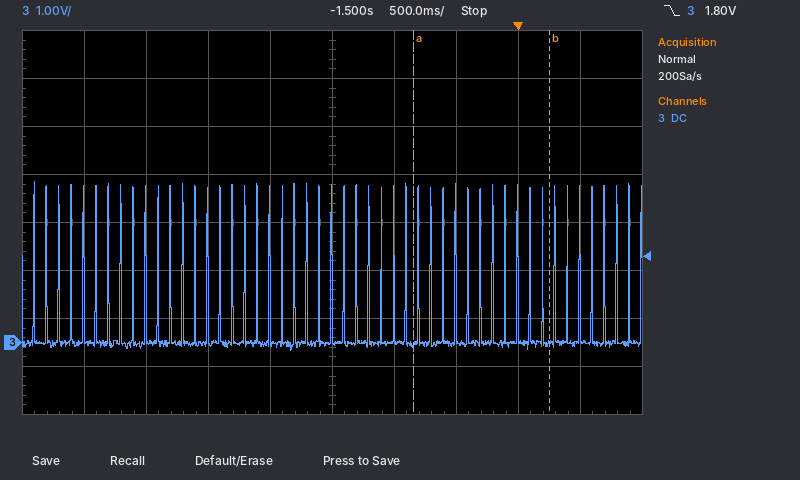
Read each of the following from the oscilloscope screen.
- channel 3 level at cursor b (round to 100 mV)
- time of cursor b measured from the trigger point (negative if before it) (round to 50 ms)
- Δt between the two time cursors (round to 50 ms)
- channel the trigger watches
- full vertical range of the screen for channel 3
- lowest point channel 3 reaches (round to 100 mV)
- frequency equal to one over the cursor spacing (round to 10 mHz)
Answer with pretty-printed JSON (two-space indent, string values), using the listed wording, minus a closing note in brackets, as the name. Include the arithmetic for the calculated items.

{
  "channel 3 level at cursor b": "0.0 V",
  "time of cursor b measured from the trigger point (negative if before it)": "+250 ms",
  "Δt between the two time cursors": "1.10 s",
  "channel the trigger watches": "channel 3",
  "full vertical range of the screen for channel 3": "8 V",
  "lowest point channel 3 reaches": "-200 mV",
  "frequency equal to one over the cursor spacing": "1 / 1.10 s ≈ 910 mHz"
}
